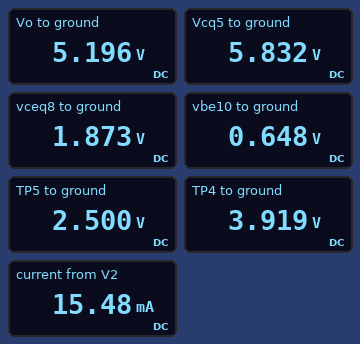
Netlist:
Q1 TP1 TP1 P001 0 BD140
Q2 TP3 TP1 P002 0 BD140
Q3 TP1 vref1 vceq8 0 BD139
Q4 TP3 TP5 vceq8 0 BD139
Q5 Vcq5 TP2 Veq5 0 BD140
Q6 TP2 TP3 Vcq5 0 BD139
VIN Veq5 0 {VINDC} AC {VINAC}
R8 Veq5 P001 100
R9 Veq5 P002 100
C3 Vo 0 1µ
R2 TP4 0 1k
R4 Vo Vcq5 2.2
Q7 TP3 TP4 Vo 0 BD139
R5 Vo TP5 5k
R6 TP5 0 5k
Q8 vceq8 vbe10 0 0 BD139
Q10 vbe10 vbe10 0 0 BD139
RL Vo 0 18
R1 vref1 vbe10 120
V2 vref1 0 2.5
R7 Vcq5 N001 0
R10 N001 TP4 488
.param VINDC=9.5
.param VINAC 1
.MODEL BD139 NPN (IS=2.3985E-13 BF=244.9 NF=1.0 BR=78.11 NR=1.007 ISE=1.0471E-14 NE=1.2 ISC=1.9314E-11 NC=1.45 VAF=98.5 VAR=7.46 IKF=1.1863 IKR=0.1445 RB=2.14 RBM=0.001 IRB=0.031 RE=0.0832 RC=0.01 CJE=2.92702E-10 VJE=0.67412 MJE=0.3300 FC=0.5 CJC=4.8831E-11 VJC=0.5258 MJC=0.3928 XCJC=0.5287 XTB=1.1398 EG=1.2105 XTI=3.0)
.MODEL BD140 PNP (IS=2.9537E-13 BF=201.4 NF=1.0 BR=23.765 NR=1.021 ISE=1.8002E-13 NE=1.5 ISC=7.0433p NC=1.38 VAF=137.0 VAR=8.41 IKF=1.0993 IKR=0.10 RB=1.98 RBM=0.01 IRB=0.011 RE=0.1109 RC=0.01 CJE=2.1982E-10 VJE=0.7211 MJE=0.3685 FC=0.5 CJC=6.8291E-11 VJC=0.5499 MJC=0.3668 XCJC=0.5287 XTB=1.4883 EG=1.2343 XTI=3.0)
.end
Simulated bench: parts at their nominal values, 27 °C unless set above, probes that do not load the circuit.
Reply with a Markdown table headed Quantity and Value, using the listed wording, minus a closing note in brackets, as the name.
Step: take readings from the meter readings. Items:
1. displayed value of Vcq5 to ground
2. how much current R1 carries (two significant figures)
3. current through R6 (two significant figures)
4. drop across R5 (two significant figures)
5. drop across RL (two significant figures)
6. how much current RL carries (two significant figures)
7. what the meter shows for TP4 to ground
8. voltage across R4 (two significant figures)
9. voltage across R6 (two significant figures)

| Quantity | Value |
|---|---|
| displayed value of Vcq5 to ground | 5.832 V |
| how much current R1 carries | 15 mA |
| current through R6 | 500 µA |
| drop across R5 | 2.7 V |
| drop across RL | 5.2 V |
| how much current RL carries | 290 mA |
| what the meter shows for TP4 to ground | 3.919 V |
| voltage across R4 | 640 mV |
| voltage across R6 | 2.5 V |
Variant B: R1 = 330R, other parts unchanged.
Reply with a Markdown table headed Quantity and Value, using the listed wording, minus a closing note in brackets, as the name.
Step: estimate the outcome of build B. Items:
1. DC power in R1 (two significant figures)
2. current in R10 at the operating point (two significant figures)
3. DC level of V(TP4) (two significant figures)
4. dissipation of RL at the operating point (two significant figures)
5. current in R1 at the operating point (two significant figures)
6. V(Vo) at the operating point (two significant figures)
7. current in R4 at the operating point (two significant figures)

| Quantity | Value |
|---|---|
| DC power in R1 | 11 mW |
| current in R10 at the operating point | 3.8 mA |
| DC level of V(TP4) | 3.8 V |
| dissipation of RL at the operating point | 1.4 W |
| current in R1 at the operating point | 5.7 mA |
| V(Vo) at the operating point | 5.1 V |
| current in R4 at the operating point | 280 mA |
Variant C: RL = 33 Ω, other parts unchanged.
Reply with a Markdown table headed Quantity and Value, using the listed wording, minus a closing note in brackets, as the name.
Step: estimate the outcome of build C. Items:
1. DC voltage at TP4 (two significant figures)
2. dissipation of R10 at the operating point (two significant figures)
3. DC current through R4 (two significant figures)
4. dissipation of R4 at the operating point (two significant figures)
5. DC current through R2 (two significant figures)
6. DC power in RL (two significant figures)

| Quantity | Value |
|---|---|
| DC voltage at TP4 | 3.7 V |
| dissipation of R10 at the operating point | 6.8 mW |
| DC current through R4 | 160 mA |
| dissipation of R4 at the operating point | 55 mW |
| DC current through R2 | 3.7 mA |
| DC power in RL | 820 mW |
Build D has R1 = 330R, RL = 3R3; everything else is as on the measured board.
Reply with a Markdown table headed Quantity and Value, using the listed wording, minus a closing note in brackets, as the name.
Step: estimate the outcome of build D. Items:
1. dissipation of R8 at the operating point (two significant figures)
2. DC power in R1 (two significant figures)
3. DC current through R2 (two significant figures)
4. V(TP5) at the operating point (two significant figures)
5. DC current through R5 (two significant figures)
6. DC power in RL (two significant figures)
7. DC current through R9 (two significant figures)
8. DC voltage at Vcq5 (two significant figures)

| Quantity | Value |
|---|---|
| dissipation of R8 at the operating point | 1.6 mW |
| DC power in R1 | 11 mW |
| DC current through R2 | 5.6 mA |
| V(TP5) at the operating point | 2.5 V |
| DC current through R5 | 500 µA |
| DC power in RL | 7.6 W |
| DC current through R9 | 4.0 mA |
| DC voltage at Vcq5 | 8.3 V |
